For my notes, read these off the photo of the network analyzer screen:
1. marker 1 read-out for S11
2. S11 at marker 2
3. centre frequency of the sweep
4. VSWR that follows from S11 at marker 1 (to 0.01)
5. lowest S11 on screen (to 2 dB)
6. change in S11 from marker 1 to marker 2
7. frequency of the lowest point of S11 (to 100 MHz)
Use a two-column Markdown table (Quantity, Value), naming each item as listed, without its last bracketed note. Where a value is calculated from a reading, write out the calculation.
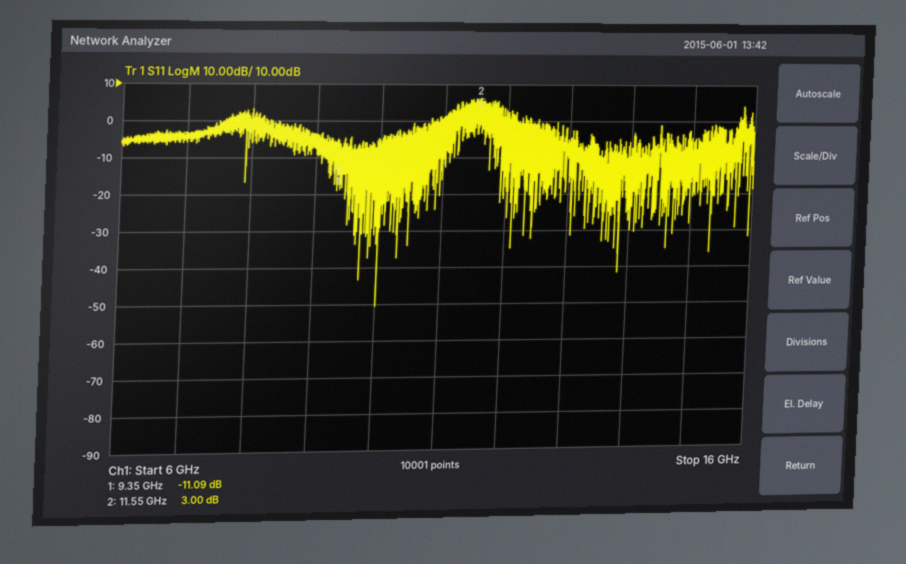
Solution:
| Quantity | Value |
|---|---|
| marker 1 read-out for S11 | -11.09 dB |
| S11 at marker 2 | 3.00 dB |
| centre frequency of the sweep | 11 GHz |
| VSWR that follows from S11 at marker 1 | (1 + 0.2789)/(1 − 0.2789) ≈ 1.77 |
| lowest S11 on screen | -50 dB |
| change in S11 from marker 1 to marker 2 | 3 − (-11.09) = 14.09 dB |
| frequency of the lowest point of S11 | 10.0 GHz |
